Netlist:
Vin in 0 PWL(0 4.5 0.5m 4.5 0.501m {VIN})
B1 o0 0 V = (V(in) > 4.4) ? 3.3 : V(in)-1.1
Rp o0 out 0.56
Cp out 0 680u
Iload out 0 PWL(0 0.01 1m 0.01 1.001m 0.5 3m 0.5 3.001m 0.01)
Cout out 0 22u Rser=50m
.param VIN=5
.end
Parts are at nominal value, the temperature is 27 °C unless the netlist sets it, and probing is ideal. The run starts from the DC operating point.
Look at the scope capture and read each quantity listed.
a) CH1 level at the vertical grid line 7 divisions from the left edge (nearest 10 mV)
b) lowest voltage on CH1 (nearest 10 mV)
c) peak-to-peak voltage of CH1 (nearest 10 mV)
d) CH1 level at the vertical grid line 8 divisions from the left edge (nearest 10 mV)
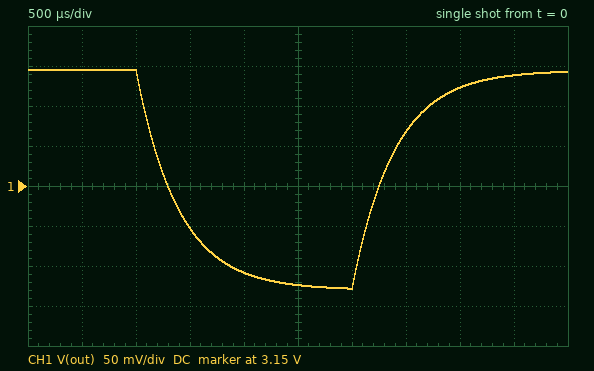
3.22 V
3.02 V
270 mV
3.27 V
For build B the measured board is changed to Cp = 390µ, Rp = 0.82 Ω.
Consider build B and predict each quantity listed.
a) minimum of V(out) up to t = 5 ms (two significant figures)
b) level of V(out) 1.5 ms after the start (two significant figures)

2.9 V
3.0 V
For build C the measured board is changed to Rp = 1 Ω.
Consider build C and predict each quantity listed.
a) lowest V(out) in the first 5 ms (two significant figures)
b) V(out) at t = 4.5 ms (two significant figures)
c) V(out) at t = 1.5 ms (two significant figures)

2.8 V
3.2 V
3.0 V
